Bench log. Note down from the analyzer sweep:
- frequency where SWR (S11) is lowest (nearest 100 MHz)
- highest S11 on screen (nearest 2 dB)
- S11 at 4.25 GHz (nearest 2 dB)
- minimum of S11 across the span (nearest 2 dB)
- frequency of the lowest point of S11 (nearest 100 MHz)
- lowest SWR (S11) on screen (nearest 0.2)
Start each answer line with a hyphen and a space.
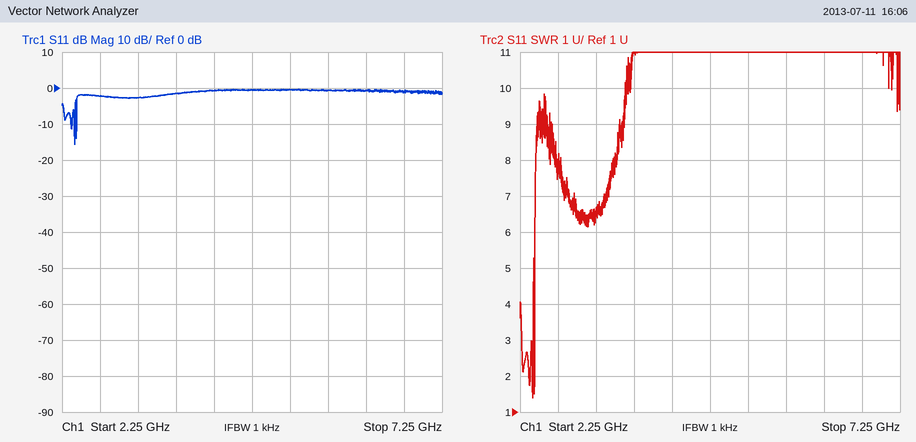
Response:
- 2.4 GHz
- 0 dB
- 0 dB
- -16 dB
- 2.4 GHz
- 1.4
